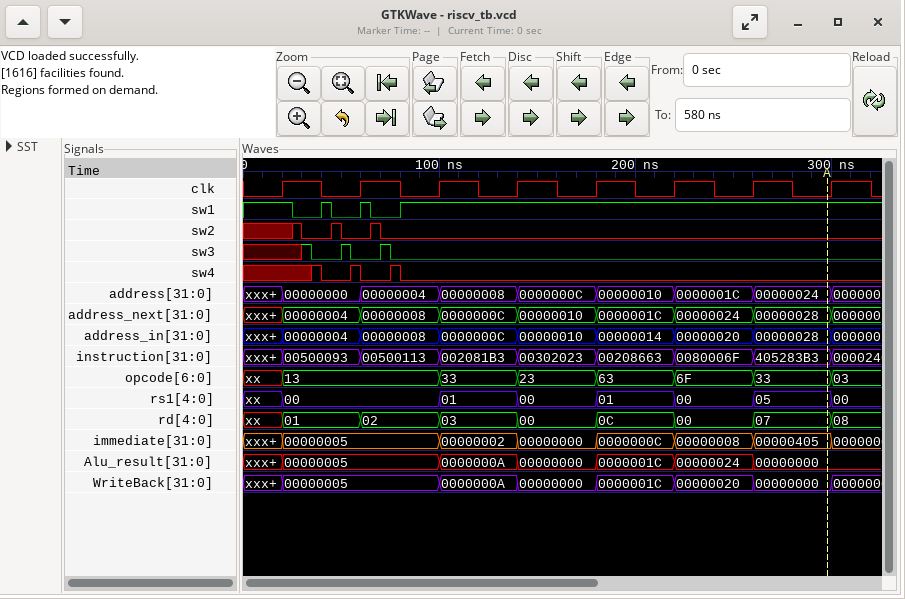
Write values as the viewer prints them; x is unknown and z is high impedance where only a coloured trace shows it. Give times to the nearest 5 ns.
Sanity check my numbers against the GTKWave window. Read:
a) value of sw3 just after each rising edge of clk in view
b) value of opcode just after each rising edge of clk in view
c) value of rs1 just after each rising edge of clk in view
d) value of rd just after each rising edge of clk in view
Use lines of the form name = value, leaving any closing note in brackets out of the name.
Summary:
value of sw3 just after each rising edge of clk in view = x 0 0 0 0 0 0 0
value of opcode just after each rising edge of clk in view = 13, 13, 33, 23, 63, 6F, 33, 03
value of rs1 just after each rising edge of clk in view = 00, 00, 01, 00, 01, 00, 05, 00
value of rd just after each rising edge of clk in view = 01, 02, 03, 00, 0C, 00, 07, 08
